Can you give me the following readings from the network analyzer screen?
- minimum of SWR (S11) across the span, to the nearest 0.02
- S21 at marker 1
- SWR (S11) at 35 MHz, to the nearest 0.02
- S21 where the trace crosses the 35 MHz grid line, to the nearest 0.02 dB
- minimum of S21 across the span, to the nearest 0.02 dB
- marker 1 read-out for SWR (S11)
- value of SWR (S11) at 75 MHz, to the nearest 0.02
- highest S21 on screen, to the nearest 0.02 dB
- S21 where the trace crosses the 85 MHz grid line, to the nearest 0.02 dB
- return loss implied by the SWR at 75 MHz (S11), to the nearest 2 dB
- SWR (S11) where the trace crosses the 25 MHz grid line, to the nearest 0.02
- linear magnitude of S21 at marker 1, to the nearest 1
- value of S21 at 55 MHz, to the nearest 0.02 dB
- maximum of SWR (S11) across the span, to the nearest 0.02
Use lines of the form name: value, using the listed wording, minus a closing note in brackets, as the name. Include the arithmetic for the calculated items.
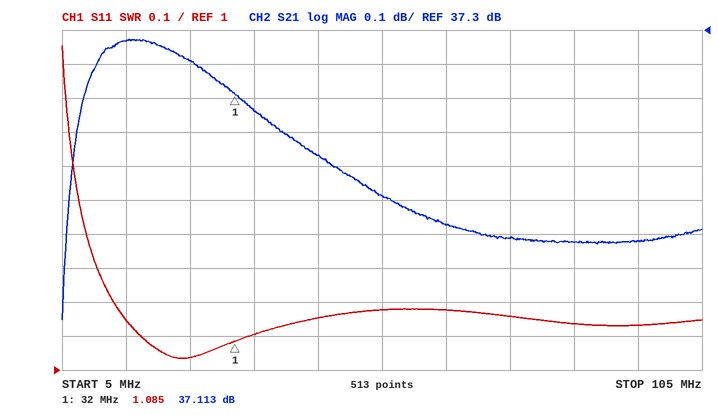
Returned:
minimum of SWR (S11) across the span, to the nearest 0.02: 1.04
S21 at marker 1: 37.113 dB
SWR (S11) at 35 MHz, to the nearest 0.02: 1.10
S21 where the trace crosses the 35 MHz grid line, to the nearest 0.02 dB: 37.06 dB
minimum of S21 across the span, to the nearest 0.02 dB: 36.44 dB
marker 1 read-out for SWR: 1.085
value of SWR (S11) at 75 MHz, to the nearest 0.02: 1.16
highest S21 on screen, to the nearest 0.02 dB: 37.28 dB
S21 where the trace crosses the 85 MHz grid line, to the nearest 0.02 dB: 36.68 dB
return loss implied by the SWR at 75 MHz (S11), to the nearest 2 dB: −20 log10((1.16 − 1)/(1.16 + 1)) ≈ 22.6 dB, so 22 dB to the nearest 2 dB
SWR (S11) where the trace crosses the 25 MHz grid line, to the nearest 0.02: 1.04
linear magnitude of S21 at marker 1, to the nearest 1: 10^(37.113/20) ≈ 72
value of S21 at 55 MHz, to the nearest 0.02 dB: 36.82 dB
maximum of SWR (S11) across the span, to the nearest 0.02: 1.96
